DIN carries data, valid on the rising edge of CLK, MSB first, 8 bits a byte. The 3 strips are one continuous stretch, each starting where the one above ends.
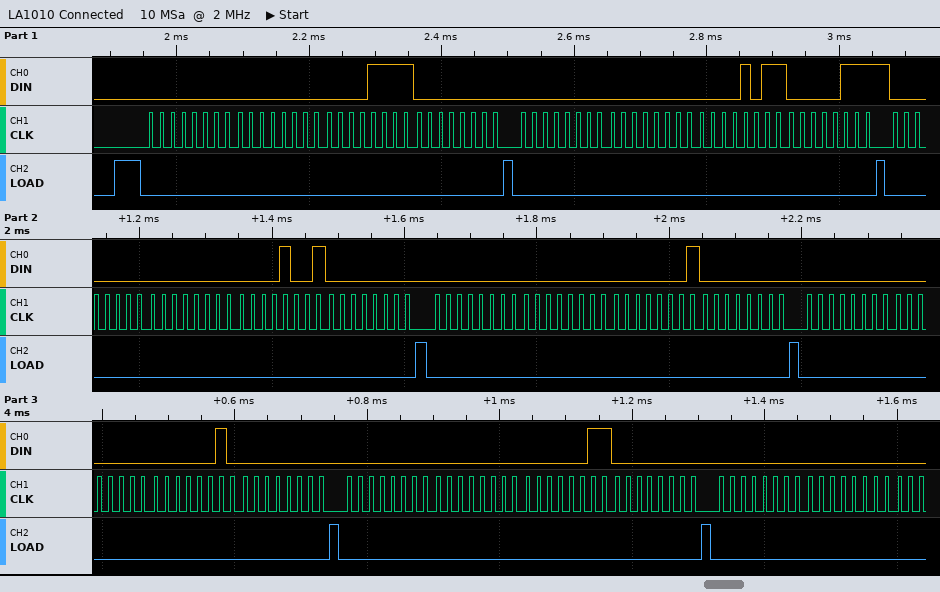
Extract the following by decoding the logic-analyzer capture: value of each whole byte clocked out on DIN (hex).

00 00 0F 00 00 00 0B 07 00 00 09 00 00 00 01 00 00 00 02 00 00 00 03 00 00 00
